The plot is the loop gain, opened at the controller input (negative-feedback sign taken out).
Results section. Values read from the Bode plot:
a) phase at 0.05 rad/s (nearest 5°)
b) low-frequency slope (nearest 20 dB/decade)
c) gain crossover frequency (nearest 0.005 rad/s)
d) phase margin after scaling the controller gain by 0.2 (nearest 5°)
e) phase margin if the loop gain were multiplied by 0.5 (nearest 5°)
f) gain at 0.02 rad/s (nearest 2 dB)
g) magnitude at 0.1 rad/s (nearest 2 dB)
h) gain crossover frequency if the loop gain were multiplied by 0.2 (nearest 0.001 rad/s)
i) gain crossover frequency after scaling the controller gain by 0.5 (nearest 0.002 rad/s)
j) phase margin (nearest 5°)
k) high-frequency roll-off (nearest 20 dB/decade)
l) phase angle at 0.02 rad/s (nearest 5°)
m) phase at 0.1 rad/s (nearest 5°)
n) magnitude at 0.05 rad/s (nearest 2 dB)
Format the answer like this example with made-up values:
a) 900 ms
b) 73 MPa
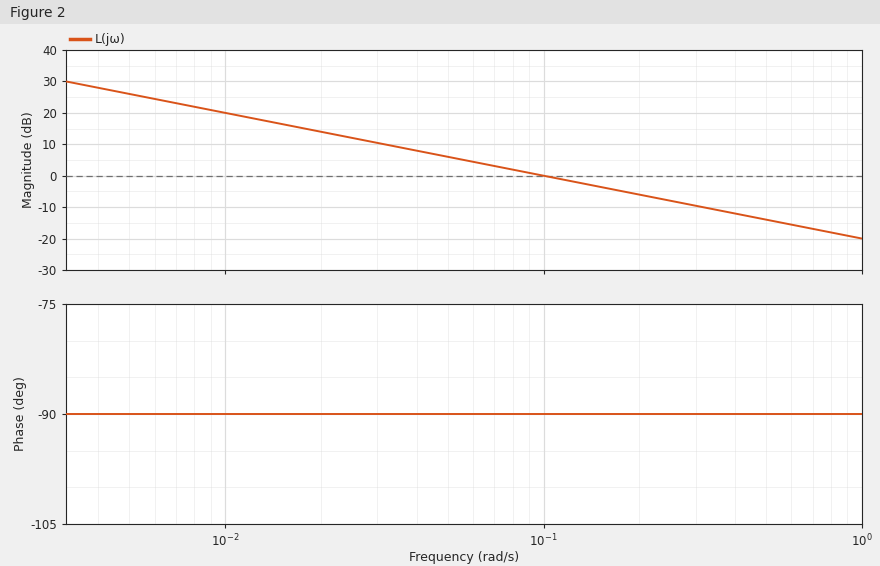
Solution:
a) -90°
b) -20 dB/decade
c) 0.100 rad/s
d) 90°
e) 90°
f) 14 dB
g) 0 dB
h) 0.020 rad/s
i) 0.050 rad/s
j) 90°
k) -20 dB/decade
l) -90°
m) -90°
n) 6 dB
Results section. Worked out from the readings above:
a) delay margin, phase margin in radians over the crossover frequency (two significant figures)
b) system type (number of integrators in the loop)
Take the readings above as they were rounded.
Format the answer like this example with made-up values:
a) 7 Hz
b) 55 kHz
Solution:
a) 16 s
b) 1
